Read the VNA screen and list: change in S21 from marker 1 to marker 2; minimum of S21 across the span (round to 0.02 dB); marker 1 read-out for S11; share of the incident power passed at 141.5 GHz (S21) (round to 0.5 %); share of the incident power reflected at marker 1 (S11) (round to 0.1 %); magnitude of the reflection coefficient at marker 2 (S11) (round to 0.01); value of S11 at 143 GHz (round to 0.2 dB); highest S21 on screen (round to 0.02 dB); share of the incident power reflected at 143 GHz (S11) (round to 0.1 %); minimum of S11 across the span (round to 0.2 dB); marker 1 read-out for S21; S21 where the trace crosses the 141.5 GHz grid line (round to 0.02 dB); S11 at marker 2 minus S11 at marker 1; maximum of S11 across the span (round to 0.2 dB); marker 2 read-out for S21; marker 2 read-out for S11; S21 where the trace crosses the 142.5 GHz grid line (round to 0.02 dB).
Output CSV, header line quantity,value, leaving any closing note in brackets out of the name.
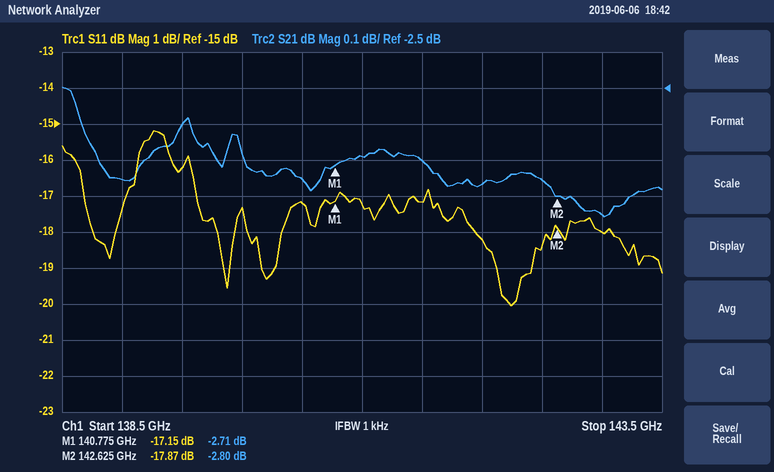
quantity,value
change in S21 from marker 1 to marker 2,-0.09 dB
minimum of S21 across the span,-2.86 dB
marker 1 read-out for S11,-17.15 dB
share of the incident power passed at 141.5 GHz (S21),53.5 %
share of the incident power reflected at marker 1 (S11),1.9 %
magnitude of the reflection coefficient at marker 2 (S11),0.13
value of S11 at 143 GHz,-18.0 dB
highest S21 on screen,-2.50 dB
share of the incident power reflected at 143 GHz (S11),1.6 %
minimum of S11 across the span,-20.0 dB
marker 1 read-out for S21,-2.71 dB
S21 where the trace crosses the 141.5 GHz grid line,-2.70 dB
S11 at marker 2 minus S11 at marker 1,-0.72 dB
maximum of S11 across the span,-15.2 dB
marker 2 read-out for S21,-2.80 dB
marker 2 read-out for S11,-17.87 dB
S21 where the trace crosses the 142.5 GHz grid line,-2.76 dB
